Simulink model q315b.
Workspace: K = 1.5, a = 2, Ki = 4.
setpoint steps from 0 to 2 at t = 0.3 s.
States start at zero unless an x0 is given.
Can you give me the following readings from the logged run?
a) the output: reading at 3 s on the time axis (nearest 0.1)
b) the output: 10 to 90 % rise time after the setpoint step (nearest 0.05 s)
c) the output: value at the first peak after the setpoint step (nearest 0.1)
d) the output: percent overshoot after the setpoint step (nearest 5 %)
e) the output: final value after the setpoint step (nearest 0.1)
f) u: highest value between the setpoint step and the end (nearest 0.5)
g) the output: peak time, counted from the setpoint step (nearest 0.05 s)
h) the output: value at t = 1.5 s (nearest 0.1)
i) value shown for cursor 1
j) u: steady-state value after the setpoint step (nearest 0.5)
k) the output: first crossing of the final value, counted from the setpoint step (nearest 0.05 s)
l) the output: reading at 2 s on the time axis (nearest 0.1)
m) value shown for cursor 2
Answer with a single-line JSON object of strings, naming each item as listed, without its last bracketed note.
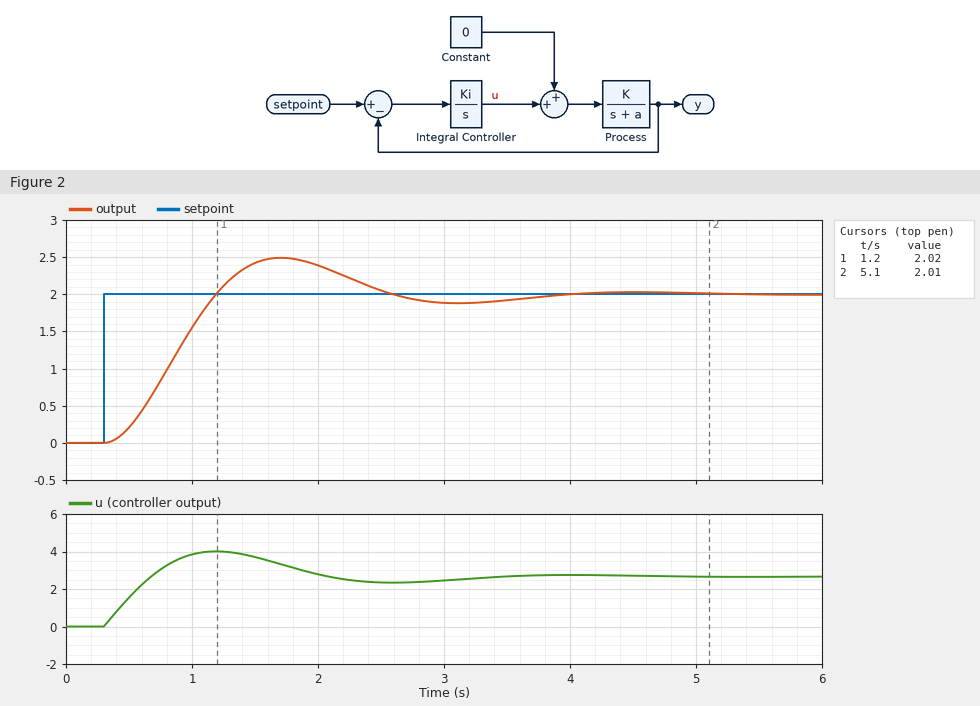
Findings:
{"the output: reading at 3 s on the time axis": "1.9", "the output: 10 to 90 % rise time after the setpoint step": "0.60 s", "the output: value at the first peak after the setpoint step": "2.5", "the output: percent overshoot after the setpoint step": "25 %", "the output: final value after the setpoint step": "2.0", "u: highest value between the setpoint step and the end": "4.0", "the output: peak time, counted from the setpoint step": "1.40 s", "the output: value at t = 1.5 s": "2.4", "value shown for cursor 1": "2.02", "u: steady-state value after the setpoint step": "2.5", "the output: first crossing of the final value, counted from the setpoint step": "0.90 s", "the output: reading at 2 s on the time axis": "2.4", "value shown for cursor 2": "2.01"}
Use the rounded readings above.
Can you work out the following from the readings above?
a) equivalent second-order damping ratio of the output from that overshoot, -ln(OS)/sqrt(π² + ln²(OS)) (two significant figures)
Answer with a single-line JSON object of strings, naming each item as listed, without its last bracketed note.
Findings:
{"equivalent second-order damping ratio of the output from that overshoot, -ln(OS)/sqrt(π² + ln²(OS))": "0.40"}
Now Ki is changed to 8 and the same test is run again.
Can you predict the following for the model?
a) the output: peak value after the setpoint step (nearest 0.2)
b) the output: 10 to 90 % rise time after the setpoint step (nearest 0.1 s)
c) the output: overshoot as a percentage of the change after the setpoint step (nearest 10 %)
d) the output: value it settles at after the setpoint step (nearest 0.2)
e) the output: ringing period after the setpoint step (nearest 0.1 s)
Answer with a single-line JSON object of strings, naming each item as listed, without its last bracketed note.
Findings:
{"the output: peak value after the setpoint step": "2.8", "the output: 10 to 90 % rise time after the setpoint step": "0.4 s", "the output: overshoot as a percentage of the change after the setpoint step": "40 %", "the output: value it settles at after the setpoint step": "2.0", "the output: ringing period after the setpoint step": "1.9 s"}
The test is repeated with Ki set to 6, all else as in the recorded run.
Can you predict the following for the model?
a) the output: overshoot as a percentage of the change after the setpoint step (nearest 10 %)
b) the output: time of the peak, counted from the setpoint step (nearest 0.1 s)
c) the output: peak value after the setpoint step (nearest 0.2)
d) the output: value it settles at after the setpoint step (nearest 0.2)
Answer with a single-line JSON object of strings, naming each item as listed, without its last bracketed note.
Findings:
{"the output: overshoot as a percentage of the change after the setpoint step": "30 %", "the output: time of the peak, counted from the setpoint step": "1.1 s", "the output: peak value after the setpoint step": "2.6", "the output: value it settles at after the setpoint step": "2.0"}
